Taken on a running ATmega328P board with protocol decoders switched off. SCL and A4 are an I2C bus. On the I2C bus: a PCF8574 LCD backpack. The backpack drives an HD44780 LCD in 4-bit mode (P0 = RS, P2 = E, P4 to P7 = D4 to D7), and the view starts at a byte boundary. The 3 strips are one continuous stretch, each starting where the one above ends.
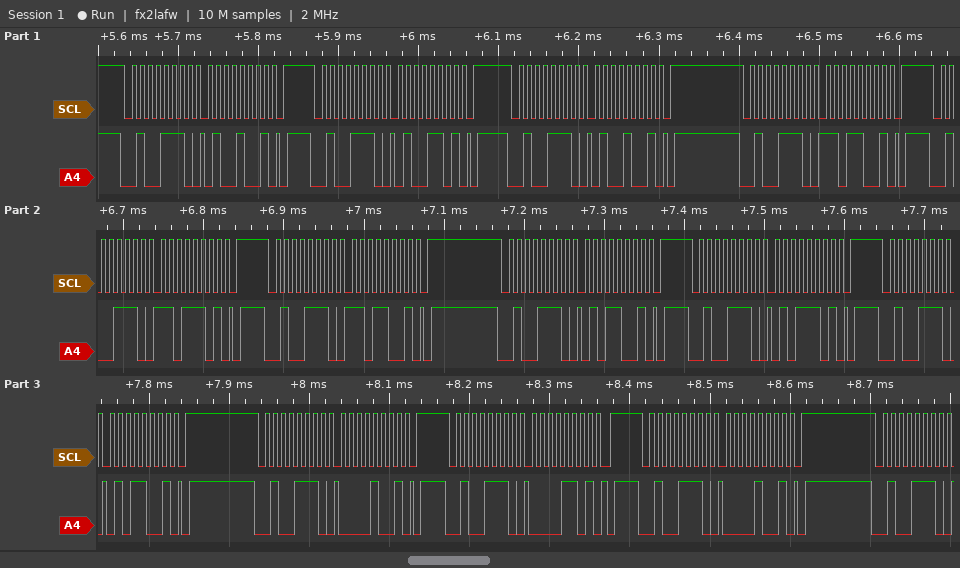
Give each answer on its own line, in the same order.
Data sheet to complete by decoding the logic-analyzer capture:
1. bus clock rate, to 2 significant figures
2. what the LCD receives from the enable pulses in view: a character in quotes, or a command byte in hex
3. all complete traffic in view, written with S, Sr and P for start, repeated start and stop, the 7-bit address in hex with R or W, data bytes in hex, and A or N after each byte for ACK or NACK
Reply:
100 kHz
'M' 'P'
S 27W A 49 A P S 27W A 4D A P S 27W A 49 A P S 27W A D9 A P S 27W A DD A P S 27W A D9 A P S 27W A 59 A P S 27W A 5D A P S 27W A 59 A P S 27W A 09 A P S 27W A 0D A P S 27W A 09 A P S 27W A
